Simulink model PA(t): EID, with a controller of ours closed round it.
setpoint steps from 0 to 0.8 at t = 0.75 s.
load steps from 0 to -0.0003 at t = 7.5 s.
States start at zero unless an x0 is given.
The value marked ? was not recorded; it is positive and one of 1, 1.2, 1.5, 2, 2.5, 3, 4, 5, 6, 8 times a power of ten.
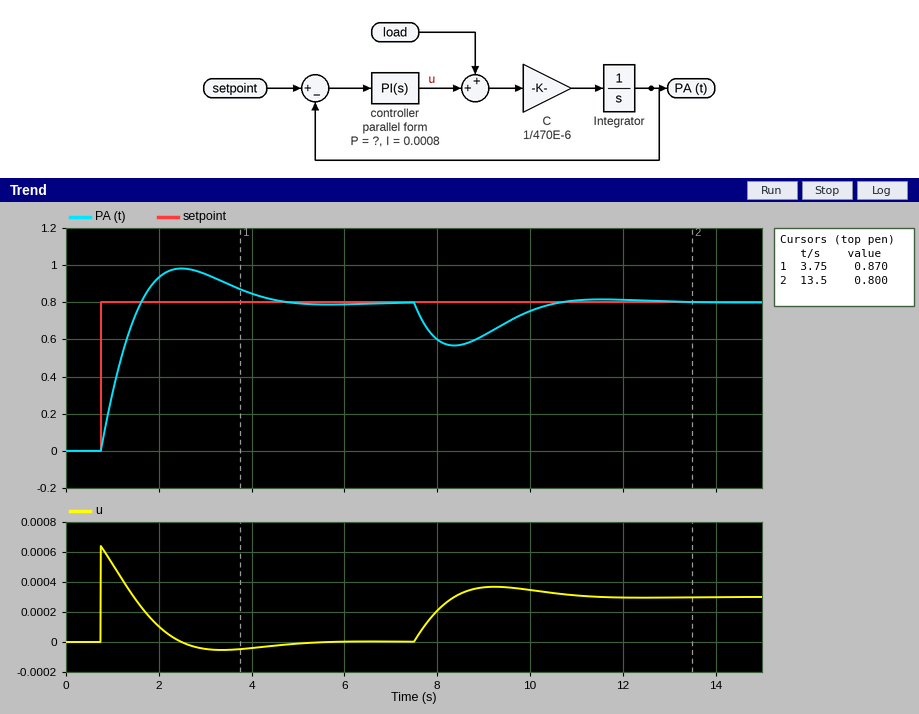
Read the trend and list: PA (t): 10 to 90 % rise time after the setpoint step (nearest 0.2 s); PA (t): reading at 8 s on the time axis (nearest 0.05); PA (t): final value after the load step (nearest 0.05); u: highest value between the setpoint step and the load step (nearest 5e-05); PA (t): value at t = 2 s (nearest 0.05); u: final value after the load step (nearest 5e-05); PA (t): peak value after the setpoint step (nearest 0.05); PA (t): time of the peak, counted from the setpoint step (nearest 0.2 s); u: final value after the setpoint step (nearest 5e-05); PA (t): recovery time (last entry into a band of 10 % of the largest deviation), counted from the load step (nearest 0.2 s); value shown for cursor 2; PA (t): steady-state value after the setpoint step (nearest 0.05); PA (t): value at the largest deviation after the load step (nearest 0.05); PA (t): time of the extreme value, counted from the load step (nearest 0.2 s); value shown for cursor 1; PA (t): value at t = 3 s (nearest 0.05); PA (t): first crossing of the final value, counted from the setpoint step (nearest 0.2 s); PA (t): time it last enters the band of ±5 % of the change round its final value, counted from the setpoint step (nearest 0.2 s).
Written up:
0.6 s
0.60
0.80
0.00065
0.95
0.00030
1.00
1.8 s
0.00000
2.8 s
0.800
0.80
0.55
0.8 s
0.870
0.95
0.8 s
3.4 s
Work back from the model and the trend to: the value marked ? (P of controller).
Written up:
0.0008
